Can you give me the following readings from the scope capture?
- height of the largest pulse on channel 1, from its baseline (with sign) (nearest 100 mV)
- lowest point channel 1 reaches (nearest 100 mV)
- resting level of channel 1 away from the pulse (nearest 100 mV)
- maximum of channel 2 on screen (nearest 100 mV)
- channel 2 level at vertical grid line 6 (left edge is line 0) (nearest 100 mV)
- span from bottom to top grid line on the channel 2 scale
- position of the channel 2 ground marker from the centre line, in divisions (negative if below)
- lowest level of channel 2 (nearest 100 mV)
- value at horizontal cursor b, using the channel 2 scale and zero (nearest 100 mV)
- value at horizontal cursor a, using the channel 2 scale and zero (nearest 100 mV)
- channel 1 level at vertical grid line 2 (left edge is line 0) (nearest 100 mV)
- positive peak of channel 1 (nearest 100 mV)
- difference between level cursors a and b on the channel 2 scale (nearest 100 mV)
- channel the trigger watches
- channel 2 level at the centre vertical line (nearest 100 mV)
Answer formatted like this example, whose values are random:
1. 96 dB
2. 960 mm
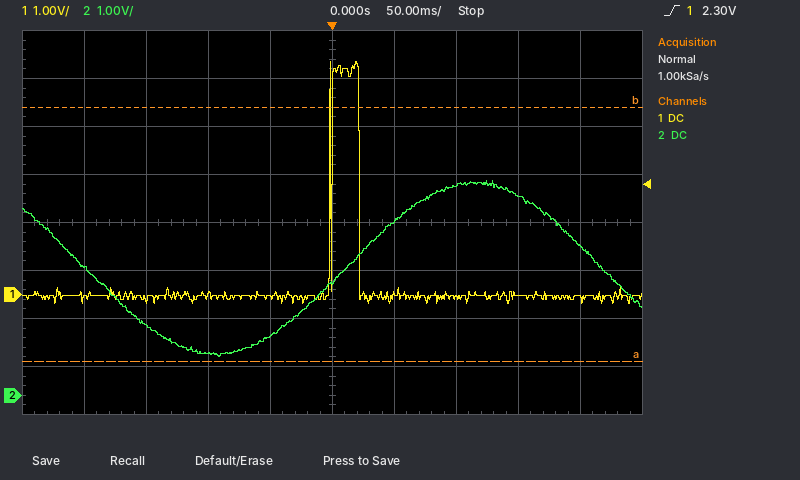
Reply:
1. +4.9 V
2. -200 mV
3. 0.0 V
4. 4.5 V
5. 3.6 V
6. 8 V
7. -3.6 div
8. 800 mV
9. 6.0 V
10. 700 mV
11. -100 mV
12. 4.9 V
13. 5.3 V
14. channel 1
15. 2.4 V
